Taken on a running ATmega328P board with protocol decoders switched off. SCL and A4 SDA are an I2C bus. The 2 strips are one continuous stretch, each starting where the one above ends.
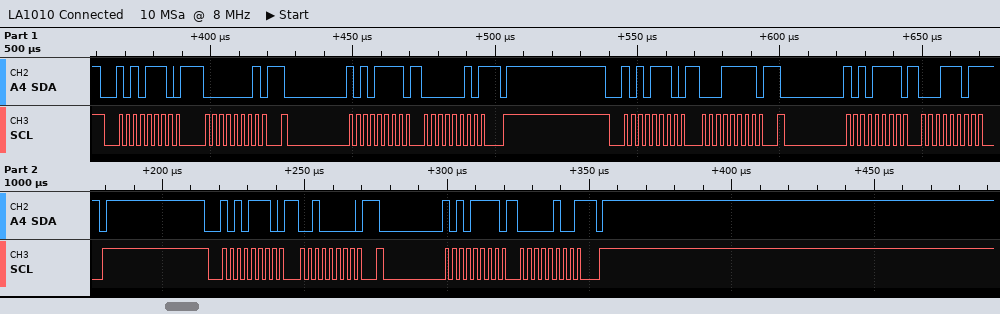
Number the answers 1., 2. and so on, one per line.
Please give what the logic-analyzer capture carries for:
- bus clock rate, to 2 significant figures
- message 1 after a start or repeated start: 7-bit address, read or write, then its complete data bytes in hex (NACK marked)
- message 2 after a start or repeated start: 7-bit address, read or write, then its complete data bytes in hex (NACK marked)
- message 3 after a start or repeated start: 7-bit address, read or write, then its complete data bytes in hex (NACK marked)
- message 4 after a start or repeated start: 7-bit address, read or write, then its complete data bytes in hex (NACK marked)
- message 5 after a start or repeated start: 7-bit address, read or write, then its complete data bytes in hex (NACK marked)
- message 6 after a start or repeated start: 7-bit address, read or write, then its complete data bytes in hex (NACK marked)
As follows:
1. 400 kHz
2. 0x57 write: 01
3. 0x57 read: 02 NACK
4. 0x57 write: 1F
5. 0x57 read: 1D NACK
6. 0x57 write: 20
7. 0x57 read: 04 NACK
